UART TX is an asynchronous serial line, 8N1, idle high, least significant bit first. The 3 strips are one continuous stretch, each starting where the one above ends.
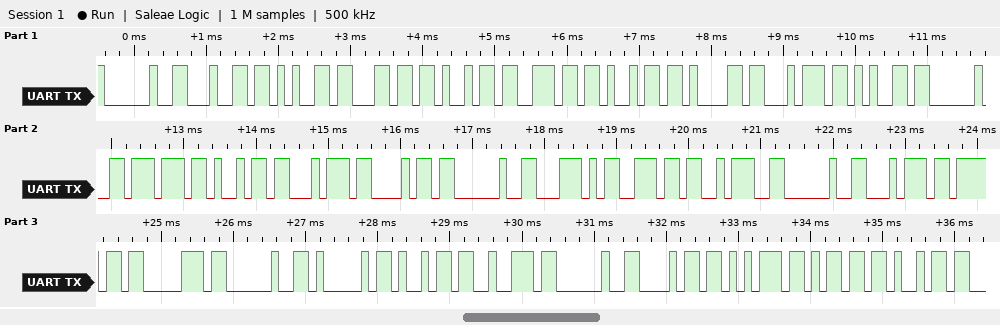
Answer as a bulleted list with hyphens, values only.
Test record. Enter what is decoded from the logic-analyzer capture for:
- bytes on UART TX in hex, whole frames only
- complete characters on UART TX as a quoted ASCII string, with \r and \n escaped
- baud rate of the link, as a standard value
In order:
- 20 64 65 6C 69 6E 69 61 74 65 20 77 69 74 68 20 5C 6E 3A 20 74 6F 70 20 41 69 72 20 68 75 6D 69
- " deliniate with \\n: top Air humi"
- 9600 baud
